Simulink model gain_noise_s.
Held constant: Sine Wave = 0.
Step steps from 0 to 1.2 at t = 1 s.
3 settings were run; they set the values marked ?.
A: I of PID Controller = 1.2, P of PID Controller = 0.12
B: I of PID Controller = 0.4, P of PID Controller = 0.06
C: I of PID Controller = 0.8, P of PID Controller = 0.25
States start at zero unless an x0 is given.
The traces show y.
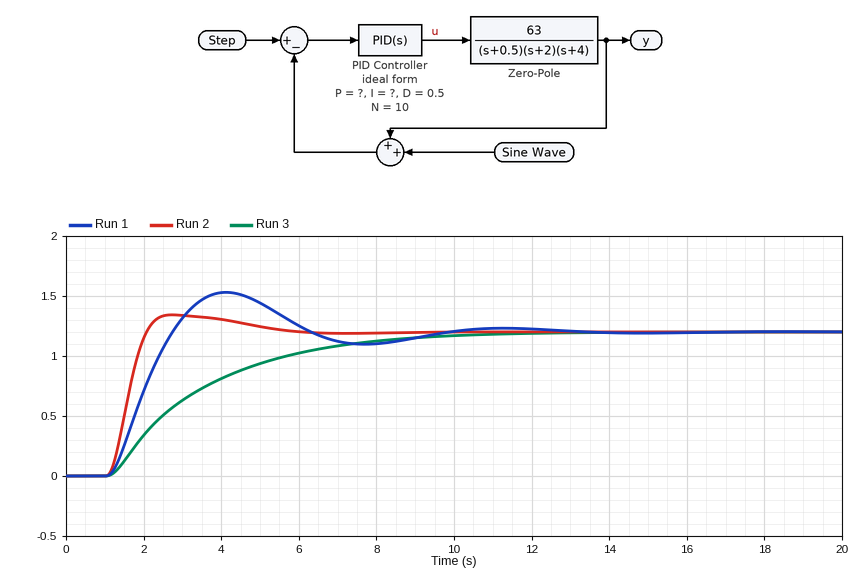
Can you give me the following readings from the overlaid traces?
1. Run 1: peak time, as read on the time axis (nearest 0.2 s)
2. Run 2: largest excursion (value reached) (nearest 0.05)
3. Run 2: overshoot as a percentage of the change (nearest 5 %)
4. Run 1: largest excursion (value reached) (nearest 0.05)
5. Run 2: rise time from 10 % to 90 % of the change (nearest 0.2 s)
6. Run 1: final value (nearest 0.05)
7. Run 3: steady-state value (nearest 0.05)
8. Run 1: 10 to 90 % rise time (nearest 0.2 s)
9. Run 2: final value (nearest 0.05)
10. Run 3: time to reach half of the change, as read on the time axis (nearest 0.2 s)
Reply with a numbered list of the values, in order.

1. 4.2 s
2. 1.35
3. 10 %
4. 1.55
5. 0.6 s
6. 1.20
7. 1.20
8. 1.2 s
9. 1.20
10. 2.8 s
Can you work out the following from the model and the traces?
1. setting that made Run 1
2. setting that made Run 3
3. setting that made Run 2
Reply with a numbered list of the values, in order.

1. A
2. B
3. C
